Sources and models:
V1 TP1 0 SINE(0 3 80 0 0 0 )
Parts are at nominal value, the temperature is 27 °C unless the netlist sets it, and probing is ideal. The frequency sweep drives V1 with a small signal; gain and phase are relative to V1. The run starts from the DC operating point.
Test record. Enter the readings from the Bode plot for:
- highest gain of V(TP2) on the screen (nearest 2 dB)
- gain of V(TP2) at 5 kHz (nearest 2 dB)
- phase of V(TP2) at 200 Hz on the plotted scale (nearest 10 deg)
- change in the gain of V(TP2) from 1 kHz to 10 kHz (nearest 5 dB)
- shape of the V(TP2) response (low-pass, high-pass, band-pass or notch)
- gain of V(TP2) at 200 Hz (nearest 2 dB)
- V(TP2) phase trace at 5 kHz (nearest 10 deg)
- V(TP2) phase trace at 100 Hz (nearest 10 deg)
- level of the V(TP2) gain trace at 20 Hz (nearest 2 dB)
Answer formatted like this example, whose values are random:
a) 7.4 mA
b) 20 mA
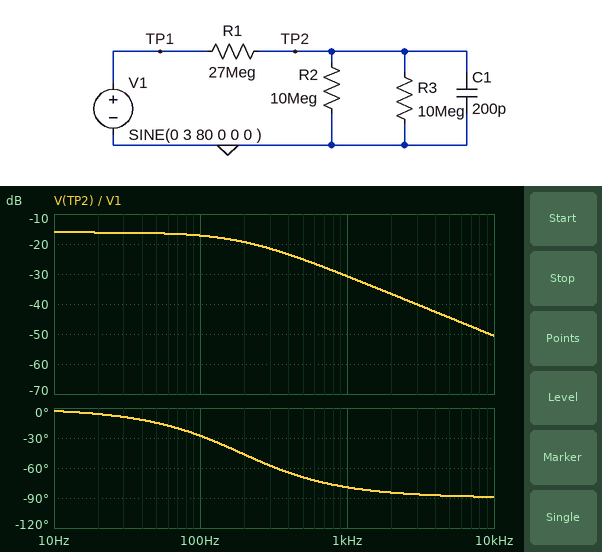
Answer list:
a) -16 dB
b) -44 dB
c) -50 deg
d) -20 dB
e) low-pass
f) -20 dB
g) -90 deg
h) -30 deg
i) -16 dB
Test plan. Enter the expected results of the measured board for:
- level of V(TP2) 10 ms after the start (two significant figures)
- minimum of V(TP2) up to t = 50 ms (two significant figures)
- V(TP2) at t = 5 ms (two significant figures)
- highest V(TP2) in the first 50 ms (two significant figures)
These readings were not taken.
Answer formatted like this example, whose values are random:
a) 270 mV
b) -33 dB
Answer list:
a) -430 mV
b) -430 mV
c) 370 mV
d) 430 mV
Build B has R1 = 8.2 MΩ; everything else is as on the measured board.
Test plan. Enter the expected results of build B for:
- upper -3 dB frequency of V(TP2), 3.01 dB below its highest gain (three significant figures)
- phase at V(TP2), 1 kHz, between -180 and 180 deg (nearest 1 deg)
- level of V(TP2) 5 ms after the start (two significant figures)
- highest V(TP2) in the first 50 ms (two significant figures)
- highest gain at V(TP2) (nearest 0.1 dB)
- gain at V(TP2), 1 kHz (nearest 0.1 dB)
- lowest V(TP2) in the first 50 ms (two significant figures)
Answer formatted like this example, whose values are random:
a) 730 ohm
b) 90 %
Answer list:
a) 256 Hz
b) -76 deg
c) 870 mV
d) 1.1 V
e) -8.4 dB
f) -20.5 dB
g) -1.1 V
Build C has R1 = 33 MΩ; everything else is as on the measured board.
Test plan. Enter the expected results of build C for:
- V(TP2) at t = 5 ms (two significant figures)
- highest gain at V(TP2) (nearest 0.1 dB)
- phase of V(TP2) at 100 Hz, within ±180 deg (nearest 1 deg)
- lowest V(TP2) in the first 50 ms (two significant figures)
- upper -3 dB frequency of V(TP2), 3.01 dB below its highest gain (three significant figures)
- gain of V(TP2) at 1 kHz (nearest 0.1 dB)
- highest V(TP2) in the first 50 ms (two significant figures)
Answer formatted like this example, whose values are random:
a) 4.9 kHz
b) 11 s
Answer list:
a) 310 mV
b) -17.6 dB
c) -29 deg
d) -360 mV
e) 183 Hz
f) -32.5 dB
g) 360 mV
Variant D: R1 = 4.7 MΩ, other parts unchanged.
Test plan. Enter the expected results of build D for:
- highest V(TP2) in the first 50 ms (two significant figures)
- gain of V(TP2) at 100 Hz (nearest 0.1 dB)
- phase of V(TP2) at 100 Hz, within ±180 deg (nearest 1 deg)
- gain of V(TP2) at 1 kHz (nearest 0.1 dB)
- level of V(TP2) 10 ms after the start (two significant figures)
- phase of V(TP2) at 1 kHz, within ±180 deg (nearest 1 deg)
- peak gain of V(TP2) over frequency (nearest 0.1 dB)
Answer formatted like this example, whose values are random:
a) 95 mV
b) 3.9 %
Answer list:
a) 1.5 V
b) -6.1 dB
c) -17 deg
d) -15.9 dB
e) -1.5 V
f) -72 deg
g) -5.8 dB
